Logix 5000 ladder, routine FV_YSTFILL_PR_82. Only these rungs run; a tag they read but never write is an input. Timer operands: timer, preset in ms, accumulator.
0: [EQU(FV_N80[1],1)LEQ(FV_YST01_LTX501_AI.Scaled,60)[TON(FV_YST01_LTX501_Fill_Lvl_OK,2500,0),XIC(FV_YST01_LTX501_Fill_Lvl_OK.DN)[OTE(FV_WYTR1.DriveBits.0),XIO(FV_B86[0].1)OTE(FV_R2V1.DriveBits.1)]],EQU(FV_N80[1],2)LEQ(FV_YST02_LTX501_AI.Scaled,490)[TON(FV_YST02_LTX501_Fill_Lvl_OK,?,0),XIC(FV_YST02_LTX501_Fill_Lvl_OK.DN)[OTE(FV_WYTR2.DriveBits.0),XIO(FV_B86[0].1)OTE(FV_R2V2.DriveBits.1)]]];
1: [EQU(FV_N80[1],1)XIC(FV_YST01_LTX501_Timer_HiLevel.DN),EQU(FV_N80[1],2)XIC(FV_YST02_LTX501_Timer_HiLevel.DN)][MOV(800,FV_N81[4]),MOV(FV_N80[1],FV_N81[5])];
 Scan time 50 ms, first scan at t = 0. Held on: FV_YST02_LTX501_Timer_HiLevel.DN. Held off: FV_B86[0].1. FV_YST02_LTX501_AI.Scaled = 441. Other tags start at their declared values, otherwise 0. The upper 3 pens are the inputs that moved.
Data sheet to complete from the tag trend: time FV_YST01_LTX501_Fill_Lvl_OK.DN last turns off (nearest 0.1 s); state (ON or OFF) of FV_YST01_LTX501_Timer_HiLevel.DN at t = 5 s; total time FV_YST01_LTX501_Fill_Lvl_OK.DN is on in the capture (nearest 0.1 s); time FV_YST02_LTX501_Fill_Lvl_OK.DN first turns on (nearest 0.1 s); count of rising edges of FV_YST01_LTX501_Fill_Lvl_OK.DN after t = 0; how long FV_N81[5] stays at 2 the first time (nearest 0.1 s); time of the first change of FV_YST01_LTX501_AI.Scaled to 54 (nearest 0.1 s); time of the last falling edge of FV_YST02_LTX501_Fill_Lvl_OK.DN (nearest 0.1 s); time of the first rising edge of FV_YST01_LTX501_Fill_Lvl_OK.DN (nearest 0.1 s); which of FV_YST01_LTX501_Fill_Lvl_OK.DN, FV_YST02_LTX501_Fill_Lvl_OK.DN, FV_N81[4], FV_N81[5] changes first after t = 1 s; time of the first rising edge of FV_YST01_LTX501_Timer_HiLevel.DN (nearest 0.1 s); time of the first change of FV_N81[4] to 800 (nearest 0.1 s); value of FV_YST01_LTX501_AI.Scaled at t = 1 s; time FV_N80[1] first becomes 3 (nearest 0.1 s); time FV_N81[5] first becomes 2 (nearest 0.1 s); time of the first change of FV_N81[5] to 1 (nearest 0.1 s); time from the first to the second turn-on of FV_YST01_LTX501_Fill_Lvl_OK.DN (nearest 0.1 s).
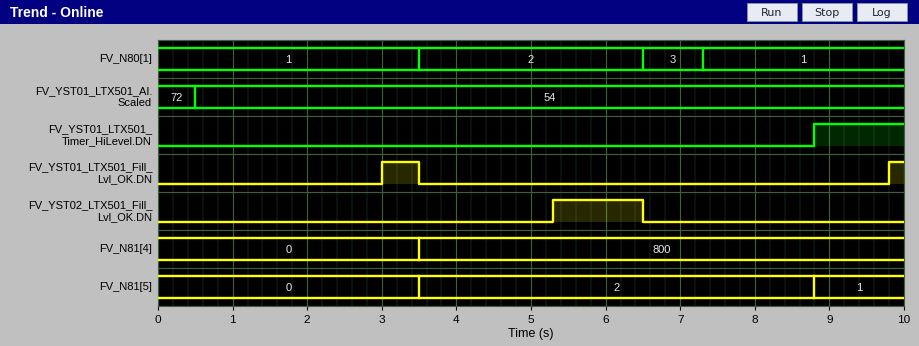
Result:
3.5 s
OFF
0.7 s
5.3 s
2
5.3 s
0.5 s
6.5 s
3.0 s
FV_YST01_LTX501_Fill_Lvl_OK.DN
8.8 s
3.5 s
54
6.5 s
3.5 s
8.8 s
6.8 s
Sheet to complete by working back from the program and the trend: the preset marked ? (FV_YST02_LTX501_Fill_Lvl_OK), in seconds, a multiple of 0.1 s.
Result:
1.8 s
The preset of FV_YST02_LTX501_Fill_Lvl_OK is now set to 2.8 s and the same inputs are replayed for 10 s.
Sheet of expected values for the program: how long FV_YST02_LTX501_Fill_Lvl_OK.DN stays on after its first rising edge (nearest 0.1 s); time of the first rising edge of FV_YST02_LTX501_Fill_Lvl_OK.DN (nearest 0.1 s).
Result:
0.2 s
6.3 s
